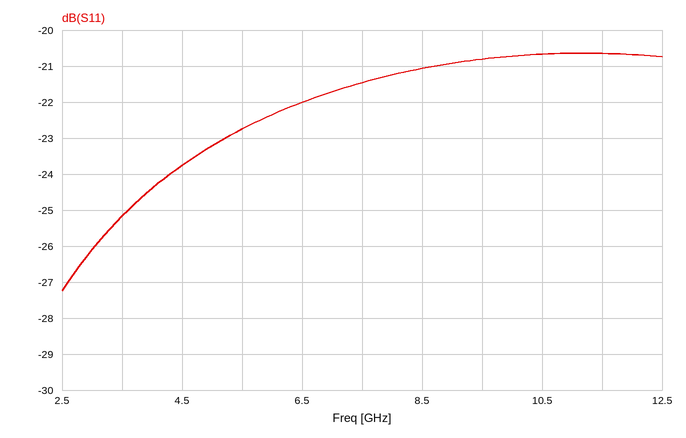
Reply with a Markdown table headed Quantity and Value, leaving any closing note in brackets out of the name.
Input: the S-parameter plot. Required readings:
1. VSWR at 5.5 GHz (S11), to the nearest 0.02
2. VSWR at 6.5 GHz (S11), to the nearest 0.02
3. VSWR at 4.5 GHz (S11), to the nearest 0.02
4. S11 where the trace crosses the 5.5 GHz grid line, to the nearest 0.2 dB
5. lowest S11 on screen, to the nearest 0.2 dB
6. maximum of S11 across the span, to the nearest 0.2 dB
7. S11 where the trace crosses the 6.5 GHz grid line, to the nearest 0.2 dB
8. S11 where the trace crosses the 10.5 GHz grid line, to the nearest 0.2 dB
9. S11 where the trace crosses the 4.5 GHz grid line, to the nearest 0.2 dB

| Quantity | Value |
|---|---|
| VSWR at 5.5 GHz (S11), to the nearest 0.02 | 1.16 |
| VSWR at 6.5 GHz (S11), to the nearest 0.02 | 1.18 |
| VSWR at 4.5 GHz (S11), to the nearest 0.02 | 1.14 |
| S11 where the trace crosses the 5.5 GHz grid line, to the nearest 0.2 dB | -22.8 dB |
| lowest S11 on screen, to the nearest 0.2 dB | -27.2 dB |
| maximum of S11 across the span, to the nearest 0.2 dB | -20.6 dB |
| S11 where the trace crosses the 6.5 GHz grid line, to the nearest 0.2 dB | -22.0 dB |
| S11 where the trace crosses the 10.5 GHz grid line, to the nearest 0.2 dB | -20.6 dB |
| S11 where the trace crosses the 4.5 GHz grid line, to the nearest 0.2 dB | -23.8 dB |
